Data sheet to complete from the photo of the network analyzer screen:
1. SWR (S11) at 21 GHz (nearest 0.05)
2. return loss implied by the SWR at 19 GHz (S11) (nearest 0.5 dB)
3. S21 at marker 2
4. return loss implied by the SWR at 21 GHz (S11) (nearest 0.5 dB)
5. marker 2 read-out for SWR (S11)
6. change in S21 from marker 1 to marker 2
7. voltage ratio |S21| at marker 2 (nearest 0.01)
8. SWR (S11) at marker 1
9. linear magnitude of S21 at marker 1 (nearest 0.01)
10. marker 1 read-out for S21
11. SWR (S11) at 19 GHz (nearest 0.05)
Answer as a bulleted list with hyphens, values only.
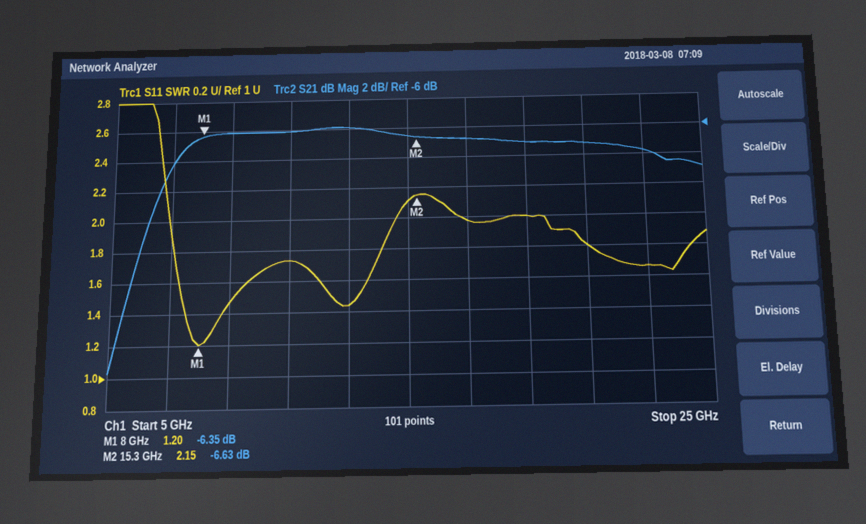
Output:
- 1.80
- 9.5 dB
- -6.63 dB
- 11.0 dB
- 2.15
- -0.28 dB
- 0.47
- 1.20
- 0.48
- -6.35 dB
- 2.00
